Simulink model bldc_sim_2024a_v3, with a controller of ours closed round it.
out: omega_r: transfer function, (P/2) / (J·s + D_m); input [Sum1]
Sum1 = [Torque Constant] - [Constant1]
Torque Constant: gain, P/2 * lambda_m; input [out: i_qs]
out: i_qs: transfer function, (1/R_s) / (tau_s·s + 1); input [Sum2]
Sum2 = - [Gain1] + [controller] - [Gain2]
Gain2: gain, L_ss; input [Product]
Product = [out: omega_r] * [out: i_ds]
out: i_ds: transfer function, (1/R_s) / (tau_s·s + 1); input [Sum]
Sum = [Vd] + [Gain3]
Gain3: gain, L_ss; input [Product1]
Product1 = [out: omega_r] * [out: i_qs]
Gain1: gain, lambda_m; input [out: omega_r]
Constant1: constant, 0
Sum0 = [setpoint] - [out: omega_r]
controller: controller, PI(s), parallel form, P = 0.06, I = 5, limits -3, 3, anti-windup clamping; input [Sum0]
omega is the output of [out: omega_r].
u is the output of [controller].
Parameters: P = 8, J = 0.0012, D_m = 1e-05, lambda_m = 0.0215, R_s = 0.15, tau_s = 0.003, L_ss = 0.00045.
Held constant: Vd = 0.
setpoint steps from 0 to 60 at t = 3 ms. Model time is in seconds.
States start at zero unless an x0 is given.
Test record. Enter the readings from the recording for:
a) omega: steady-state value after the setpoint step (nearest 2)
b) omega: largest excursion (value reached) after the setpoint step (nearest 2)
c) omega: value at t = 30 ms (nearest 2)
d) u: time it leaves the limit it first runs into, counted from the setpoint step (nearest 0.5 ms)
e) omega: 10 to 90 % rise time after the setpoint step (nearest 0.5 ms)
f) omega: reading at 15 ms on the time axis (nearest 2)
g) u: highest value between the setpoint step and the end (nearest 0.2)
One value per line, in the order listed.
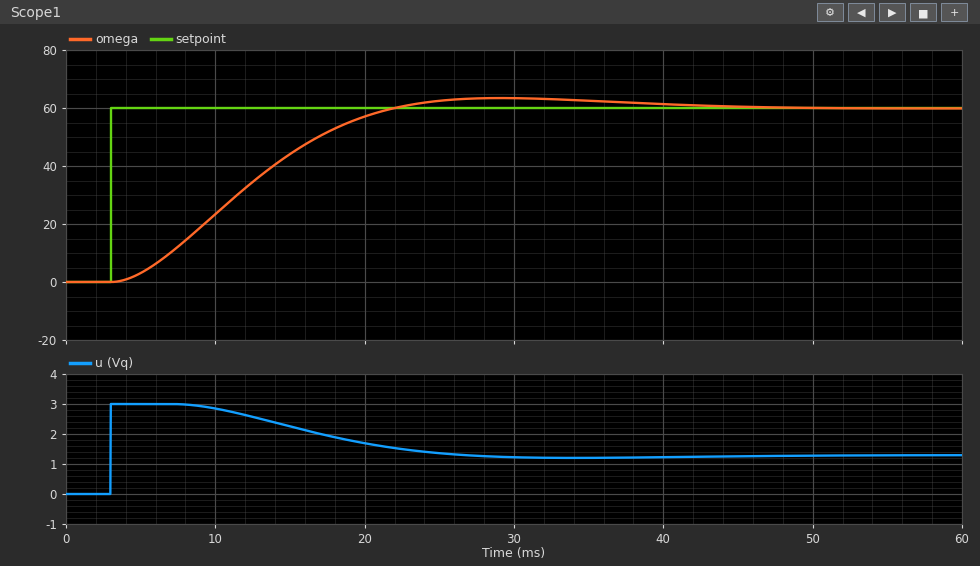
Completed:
60
64
64
5.5 ms
12.5 ms
44
3.0
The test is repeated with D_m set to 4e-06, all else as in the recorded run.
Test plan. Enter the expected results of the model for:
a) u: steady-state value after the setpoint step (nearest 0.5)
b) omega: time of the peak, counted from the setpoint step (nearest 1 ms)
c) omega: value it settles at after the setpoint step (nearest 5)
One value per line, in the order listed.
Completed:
1.5
26 ms
60
